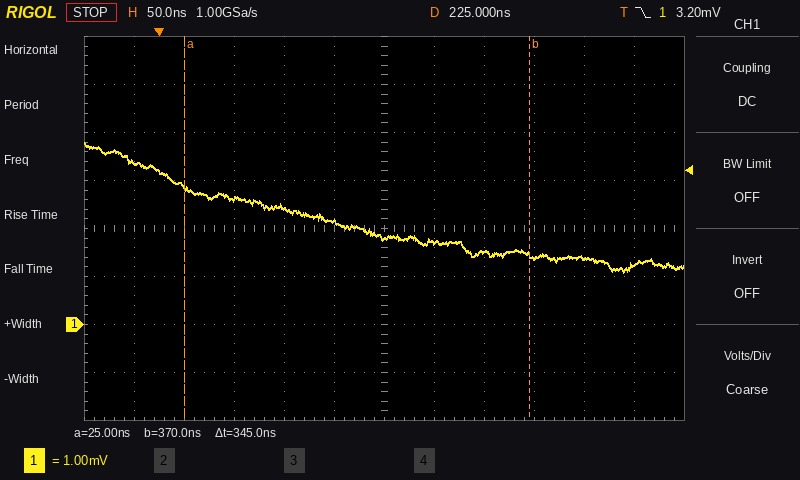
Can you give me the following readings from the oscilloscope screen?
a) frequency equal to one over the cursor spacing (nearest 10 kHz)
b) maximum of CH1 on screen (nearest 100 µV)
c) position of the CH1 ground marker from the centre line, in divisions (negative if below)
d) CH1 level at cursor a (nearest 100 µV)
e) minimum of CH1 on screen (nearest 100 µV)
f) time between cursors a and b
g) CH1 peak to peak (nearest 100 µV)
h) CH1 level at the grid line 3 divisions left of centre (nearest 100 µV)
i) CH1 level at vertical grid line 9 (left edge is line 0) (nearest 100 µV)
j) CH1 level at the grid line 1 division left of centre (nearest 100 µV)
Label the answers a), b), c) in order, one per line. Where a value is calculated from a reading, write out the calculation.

a) 1 / 345 ns ≈ 2.90 MHz
b) 3.8 mV
c) -2.0 div
d) 2.9 mV
e) 1.1 mV
f) 345 ns
g) 3.8 mV − (1.1 mV) = 2.7 mV
h) 2.6 mV
i) 1.4 mV
j) 2.1 mV
